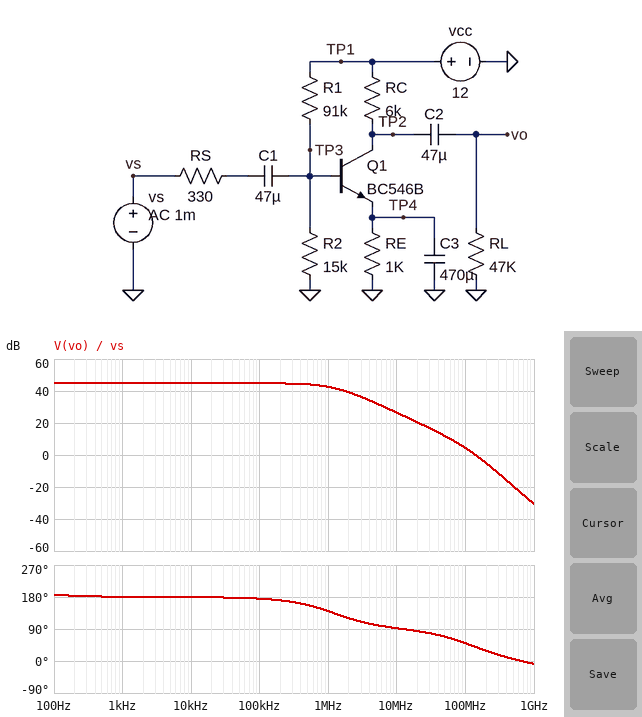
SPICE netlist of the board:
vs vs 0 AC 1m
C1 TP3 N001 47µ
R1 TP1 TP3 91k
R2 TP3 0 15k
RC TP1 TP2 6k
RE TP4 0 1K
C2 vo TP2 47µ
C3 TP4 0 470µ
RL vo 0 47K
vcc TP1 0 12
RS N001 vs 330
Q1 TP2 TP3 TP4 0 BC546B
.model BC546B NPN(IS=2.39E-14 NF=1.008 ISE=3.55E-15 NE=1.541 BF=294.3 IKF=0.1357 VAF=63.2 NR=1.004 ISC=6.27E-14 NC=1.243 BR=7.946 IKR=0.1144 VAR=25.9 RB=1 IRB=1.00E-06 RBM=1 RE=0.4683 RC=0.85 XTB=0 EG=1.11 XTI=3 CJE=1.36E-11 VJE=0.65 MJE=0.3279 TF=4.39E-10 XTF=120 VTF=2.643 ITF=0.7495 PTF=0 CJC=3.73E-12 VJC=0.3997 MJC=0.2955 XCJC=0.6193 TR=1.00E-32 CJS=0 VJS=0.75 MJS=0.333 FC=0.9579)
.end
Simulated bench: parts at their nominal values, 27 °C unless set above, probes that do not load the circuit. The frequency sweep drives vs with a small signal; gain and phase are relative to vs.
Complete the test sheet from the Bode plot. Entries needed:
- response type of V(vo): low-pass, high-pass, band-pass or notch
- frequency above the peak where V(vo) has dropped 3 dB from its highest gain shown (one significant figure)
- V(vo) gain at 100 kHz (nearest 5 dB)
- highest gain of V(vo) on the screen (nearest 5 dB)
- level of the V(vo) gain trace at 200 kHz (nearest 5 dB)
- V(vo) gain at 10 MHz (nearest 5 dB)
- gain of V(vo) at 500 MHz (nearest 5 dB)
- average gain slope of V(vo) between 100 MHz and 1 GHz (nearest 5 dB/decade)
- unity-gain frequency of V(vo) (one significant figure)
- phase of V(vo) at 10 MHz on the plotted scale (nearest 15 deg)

low-pass
1 MHz
45 dB
45 dB
45 dB
25 dB
-20 dB
-35 dB/decade
100 MHz
90 deg
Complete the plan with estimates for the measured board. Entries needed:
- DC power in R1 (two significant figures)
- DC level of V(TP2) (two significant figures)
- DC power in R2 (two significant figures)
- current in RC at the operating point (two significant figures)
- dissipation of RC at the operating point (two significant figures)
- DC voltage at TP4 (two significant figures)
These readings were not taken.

1.2 mW
5.9 V
180 µW
1.0 mA
6.2 mW
1.0 V
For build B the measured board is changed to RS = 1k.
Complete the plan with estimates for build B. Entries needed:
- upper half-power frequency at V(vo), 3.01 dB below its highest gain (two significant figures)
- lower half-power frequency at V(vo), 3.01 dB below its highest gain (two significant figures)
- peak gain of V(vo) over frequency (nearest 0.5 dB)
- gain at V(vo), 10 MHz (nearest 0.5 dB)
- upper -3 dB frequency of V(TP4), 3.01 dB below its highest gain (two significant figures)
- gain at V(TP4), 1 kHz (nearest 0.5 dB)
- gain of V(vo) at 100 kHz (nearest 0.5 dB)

470 kHz
11 Hz
44.0 dB
17.0 dB
12 Hz
-40.0 dB
43.5 dB
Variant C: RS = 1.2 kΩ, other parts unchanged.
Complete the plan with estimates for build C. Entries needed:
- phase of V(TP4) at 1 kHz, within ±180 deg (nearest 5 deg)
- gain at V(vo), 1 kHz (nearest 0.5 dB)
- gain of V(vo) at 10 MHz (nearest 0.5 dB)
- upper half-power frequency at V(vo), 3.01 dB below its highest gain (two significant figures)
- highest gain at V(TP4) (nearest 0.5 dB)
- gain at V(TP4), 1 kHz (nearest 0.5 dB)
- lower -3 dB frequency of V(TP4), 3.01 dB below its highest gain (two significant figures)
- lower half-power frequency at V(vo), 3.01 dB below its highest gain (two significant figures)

-90 deg
43.5 dB
15.5 dB
410 kHz
-1.5 dB
-40.5 dB
230 mHz
11 Hz
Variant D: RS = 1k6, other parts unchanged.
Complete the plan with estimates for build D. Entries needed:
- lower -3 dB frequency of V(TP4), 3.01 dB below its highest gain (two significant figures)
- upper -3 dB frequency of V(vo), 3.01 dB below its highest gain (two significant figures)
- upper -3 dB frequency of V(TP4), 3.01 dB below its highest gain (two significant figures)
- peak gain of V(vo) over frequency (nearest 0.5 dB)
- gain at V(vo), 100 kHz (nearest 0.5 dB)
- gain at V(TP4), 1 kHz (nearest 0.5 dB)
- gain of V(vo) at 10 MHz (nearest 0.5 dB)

230 mHz
330 kHz
11 Hz
43.0 dB
42.5 dB
-41.0 dB
13.0 dB
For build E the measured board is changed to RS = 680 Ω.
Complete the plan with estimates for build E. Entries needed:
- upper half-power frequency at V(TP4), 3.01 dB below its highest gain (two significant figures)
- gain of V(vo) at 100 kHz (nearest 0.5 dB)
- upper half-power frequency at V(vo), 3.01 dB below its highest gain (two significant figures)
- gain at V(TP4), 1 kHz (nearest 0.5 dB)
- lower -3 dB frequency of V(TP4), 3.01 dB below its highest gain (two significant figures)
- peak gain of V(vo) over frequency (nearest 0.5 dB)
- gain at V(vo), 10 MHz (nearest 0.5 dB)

12 Hz
44.0 dB
650 kHz
-39.5 dB
240 mHz
44.5 dB
20.5 dB
